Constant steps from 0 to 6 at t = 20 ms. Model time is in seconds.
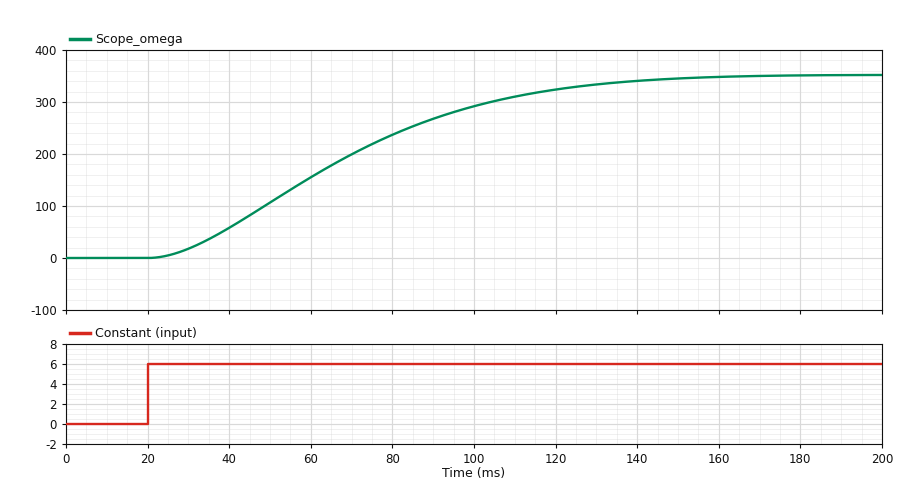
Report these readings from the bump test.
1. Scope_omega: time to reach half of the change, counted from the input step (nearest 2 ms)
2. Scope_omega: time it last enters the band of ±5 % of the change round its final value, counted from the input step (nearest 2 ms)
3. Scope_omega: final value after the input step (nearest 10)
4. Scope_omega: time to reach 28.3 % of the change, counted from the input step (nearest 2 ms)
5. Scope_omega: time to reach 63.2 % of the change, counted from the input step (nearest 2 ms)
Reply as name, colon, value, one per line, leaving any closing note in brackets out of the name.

Scope_omega: time to reach half of the change, counted from the input step: 44 ms
Scope_omega: time it last enters the band of ±5 % of the change round its final value, counted from the input step: 110 ms
Scope_omega: final value after the input step: 350
Scope_omega: time to reach 28.3 % of the change, counted from the input step: 28 ms
Scope_omega: time to reach 63.2 % of the change, counted from the input step: 56 ms
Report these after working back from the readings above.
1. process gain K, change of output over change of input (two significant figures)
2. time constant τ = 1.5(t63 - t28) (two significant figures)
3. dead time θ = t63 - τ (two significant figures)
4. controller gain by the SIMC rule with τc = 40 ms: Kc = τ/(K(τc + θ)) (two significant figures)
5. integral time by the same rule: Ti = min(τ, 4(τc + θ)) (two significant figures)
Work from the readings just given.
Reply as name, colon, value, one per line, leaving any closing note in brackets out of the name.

process gain K, change of output over change of input: 58
time constant τ = 1.5(t63 - t28): 42 ms
dead time θ = t63 - τ: 14 ms
controller gain by the SIMC rule with τc = 40 ms: Kc = τ/(K(τc + θ)): 0.013
integral time by the same rule: Ti = min(τ, 4(τc + θ)): 42 ms
